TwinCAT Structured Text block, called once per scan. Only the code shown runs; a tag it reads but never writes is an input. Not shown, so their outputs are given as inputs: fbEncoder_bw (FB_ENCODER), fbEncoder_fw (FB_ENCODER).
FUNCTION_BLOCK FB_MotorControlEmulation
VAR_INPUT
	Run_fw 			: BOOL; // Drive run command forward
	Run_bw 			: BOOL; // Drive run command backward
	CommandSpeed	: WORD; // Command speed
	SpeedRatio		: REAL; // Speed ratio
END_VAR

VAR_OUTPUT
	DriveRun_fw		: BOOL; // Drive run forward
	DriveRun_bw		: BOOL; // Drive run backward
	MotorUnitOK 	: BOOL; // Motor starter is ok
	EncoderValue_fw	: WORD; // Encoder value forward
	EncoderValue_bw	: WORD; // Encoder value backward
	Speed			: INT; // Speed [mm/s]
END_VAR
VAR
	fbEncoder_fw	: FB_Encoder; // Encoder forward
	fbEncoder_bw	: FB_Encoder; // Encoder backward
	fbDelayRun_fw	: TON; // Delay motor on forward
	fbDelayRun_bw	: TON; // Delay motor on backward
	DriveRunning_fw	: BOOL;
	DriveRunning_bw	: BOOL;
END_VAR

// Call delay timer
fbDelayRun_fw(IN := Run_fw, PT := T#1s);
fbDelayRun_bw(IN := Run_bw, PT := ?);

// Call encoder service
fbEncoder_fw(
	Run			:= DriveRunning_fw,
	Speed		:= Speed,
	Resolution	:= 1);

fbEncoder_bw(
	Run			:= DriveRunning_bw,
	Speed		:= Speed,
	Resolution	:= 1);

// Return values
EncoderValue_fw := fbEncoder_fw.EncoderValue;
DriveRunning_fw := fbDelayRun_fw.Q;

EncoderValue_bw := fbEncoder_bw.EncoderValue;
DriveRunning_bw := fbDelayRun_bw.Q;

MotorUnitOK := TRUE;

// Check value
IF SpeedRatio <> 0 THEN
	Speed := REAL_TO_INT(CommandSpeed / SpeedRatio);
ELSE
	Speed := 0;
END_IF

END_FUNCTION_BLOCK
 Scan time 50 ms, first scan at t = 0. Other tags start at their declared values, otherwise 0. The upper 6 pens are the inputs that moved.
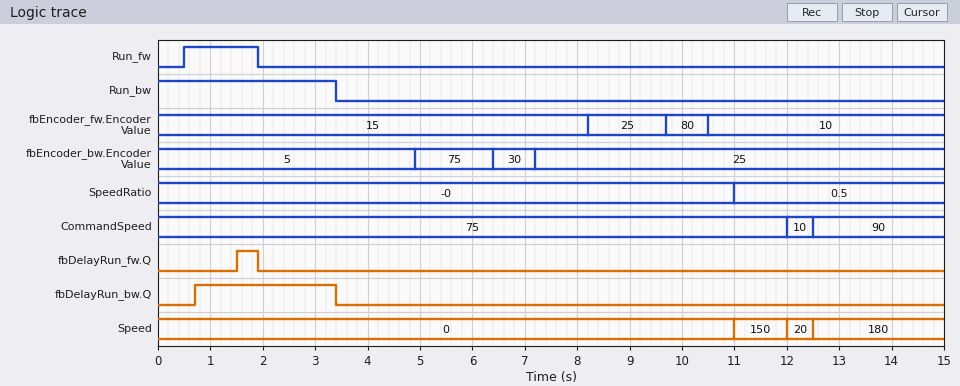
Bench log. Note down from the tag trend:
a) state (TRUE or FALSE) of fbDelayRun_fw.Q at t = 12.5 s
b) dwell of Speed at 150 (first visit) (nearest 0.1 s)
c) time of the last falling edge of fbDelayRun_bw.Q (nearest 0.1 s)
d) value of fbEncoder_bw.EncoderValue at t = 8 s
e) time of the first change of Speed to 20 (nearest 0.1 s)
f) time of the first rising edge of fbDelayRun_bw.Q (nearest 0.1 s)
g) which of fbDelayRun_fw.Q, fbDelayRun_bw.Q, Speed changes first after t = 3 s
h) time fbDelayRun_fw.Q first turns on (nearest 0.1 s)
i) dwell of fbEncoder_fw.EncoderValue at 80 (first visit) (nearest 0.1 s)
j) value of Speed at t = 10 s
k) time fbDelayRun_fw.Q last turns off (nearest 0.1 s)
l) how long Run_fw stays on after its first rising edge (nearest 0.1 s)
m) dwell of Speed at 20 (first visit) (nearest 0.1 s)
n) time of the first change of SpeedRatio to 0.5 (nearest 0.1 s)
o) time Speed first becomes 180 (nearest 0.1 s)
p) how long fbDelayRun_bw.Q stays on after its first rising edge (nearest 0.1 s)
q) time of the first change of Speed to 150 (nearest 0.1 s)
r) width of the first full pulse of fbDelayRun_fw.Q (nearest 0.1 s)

FALSE
1.0 s
3.4 s
25
12.0 s
0.7 s
fbDelayRun_bw.Q
1.5 s
0.8 s
0
1.9 s
1.4 s
0.5 s
11.0 s
12.5 s
2.7 s
11.0 s
0.4 s
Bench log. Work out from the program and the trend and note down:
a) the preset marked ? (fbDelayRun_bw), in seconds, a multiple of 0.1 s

0.7 s
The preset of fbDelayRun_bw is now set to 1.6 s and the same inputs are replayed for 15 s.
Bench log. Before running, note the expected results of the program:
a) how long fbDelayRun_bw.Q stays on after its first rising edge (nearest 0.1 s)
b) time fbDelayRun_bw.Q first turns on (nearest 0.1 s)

1.8 s
1.6 s
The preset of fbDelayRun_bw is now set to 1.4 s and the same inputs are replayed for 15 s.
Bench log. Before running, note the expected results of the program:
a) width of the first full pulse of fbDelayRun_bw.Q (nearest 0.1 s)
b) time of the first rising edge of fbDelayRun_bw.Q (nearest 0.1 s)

2.0 s
1.4 s
